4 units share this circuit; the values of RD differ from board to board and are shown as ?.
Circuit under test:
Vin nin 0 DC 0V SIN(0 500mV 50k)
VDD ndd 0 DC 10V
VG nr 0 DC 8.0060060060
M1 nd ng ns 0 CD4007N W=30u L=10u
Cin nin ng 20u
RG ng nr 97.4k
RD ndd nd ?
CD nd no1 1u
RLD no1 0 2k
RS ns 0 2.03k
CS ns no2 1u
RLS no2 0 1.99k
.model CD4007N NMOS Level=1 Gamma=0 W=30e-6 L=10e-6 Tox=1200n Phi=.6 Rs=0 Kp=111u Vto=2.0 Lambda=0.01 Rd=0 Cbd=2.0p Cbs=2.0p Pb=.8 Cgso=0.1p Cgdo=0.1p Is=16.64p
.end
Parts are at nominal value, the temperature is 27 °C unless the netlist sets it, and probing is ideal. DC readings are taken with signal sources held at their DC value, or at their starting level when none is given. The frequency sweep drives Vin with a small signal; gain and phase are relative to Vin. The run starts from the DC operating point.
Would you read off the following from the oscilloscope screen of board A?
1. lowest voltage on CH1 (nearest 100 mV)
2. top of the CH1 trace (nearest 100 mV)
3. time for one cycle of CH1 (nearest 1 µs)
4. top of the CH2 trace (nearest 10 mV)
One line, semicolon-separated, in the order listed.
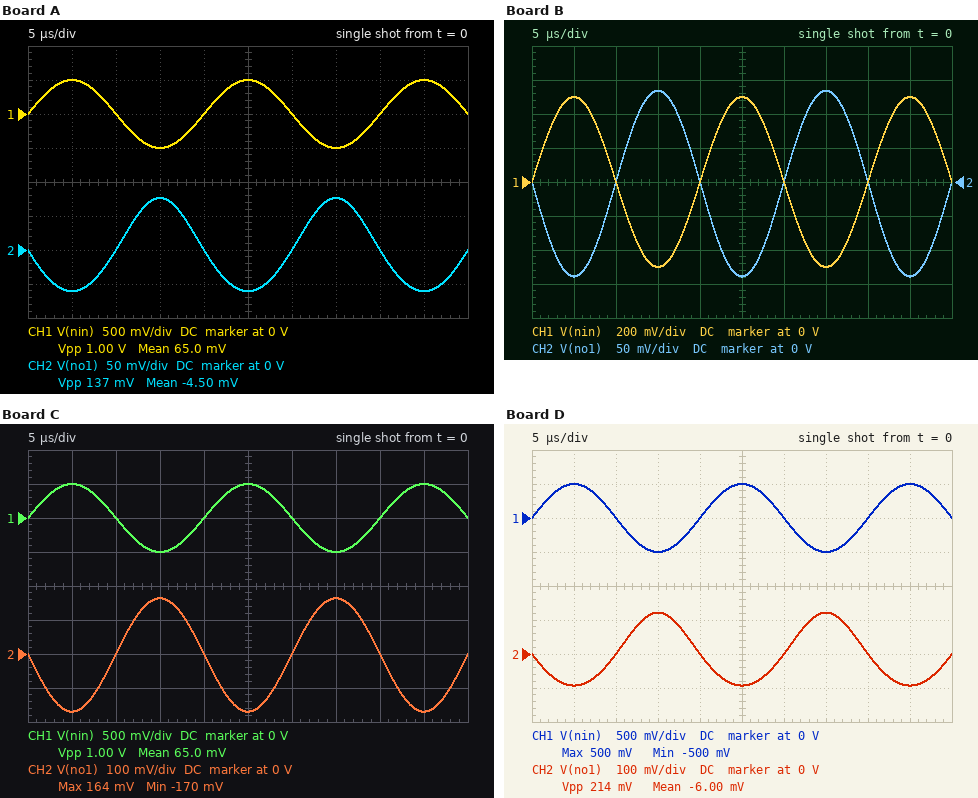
-500 mV; 500 mV; 20 µs; 80 mV
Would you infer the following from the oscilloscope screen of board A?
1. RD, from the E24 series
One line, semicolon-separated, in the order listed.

6.2 kΩ
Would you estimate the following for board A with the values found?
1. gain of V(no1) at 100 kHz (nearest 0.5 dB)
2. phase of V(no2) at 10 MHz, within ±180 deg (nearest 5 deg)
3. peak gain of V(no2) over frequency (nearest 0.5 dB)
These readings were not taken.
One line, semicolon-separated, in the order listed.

-17.5 dB; 0 deg; -20.5 dB
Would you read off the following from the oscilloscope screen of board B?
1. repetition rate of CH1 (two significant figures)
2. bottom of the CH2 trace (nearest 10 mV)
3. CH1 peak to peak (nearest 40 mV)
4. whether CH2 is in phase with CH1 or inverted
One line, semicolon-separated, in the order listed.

50 kHz; -140 mV; 1.00 V; inverted
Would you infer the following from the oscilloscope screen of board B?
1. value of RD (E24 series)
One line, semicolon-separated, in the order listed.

750 Ω
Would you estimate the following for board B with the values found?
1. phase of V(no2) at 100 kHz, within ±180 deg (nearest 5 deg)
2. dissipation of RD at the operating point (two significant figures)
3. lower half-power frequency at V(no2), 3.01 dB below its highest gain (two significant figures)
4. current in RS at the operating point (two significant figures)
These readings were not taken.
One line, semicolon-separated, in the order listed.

0 deg; 1.7 mW; 60 Hz; 1.5 mA
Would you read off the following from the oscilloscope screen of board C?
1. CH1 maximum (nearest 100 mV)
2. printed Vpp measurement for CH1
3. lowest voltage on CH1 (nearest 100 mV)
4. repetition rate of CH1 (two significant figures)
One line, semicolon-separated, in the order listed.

500 mV; 1.00 V; -500 mV; 50 kHz
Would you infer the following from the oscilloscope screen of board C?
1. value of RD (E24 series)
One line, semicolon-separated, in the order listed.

1 kΩ
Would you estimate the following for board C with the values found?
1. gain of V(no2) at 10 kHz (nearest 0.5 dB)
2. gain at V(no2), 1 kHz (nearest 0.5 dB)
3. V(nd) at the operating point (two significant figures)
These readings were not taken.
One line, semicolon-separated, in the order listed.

-6.0 dB; -6.0 dB; 8.5 V
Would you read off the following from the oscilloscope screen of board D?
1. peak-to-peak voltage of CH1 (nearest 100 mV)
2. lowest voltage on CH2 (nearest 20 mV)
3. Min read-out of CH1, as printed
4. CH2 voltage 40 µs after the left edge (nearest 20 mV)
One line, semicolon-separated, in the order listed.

1.0 V; -100 mV; -500 mV; 0 V
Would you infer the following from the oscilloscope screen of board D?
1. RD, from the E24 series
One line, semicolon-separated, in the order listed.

4.7 kΩ
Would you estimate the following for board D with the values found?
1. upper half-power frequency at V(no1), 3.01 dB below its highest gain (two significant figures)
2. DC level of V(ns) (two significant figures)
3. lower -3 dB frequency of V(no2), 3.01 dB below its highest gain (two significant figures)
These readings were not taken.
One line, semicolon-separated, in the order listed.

380 MHz; 2.6 V; 71 Hz
